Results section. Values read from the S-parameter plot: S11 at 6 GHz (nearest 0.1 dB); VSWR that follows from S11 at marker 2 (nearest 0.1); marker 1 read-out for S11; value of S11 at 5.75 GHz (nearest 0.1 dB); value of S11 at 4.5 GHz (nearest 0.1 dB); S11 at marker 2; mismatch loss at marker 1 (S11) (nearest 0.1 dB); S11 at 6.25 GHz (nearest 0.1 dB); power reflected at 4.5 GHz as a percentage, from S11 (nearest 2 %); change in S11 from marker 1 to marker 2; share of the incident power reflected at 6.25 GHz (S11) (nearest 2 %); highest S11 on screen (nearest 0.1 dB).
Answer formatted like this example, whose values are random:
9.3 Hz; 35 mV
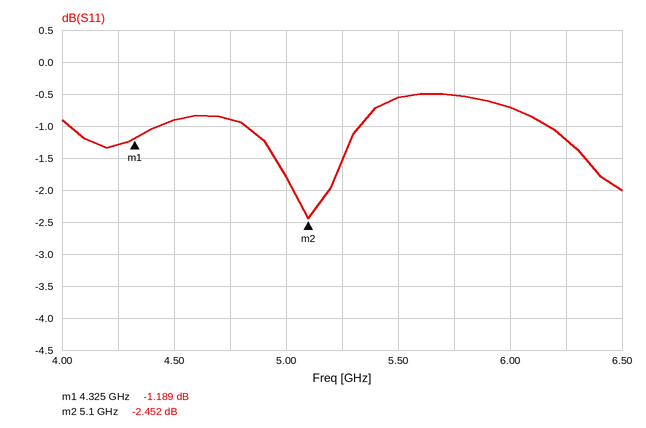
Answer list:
-0.7 dB; 7.1; -1.189 dB; -0.5 dB; -0.9 dB; -2.452 dB; 6.2 dB; -1.2 dB; 82 %; -1.263 dB; 76 %; -0.5 dB
